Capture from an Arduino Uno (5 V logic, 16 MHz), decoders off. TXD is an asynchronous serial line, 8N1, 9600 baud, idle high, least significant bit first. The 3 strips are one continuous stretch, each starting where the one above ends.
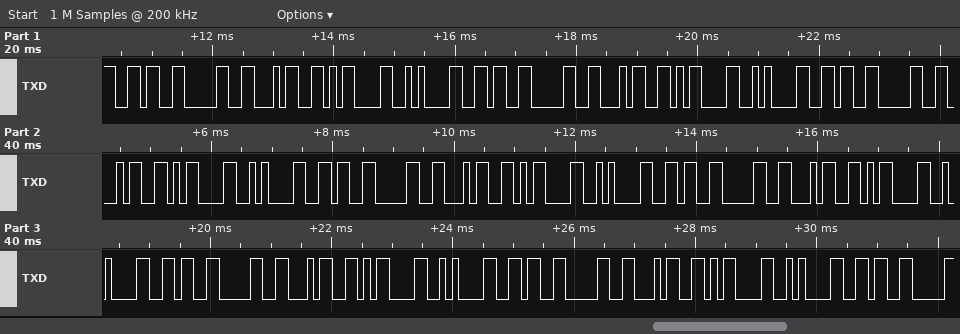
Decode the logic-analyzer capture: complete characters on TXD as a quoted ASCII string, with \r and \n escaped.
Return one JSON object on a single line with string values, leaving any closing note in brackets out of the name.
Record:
{"complete characters on TXD as a quoted ASCII string, with \\r and \\n escaped": "\"604\\r\\n604\\r\\n604\\r\\n604\\r\\n604\\r\\n604\\r\\n604\\r\\n6\""}
